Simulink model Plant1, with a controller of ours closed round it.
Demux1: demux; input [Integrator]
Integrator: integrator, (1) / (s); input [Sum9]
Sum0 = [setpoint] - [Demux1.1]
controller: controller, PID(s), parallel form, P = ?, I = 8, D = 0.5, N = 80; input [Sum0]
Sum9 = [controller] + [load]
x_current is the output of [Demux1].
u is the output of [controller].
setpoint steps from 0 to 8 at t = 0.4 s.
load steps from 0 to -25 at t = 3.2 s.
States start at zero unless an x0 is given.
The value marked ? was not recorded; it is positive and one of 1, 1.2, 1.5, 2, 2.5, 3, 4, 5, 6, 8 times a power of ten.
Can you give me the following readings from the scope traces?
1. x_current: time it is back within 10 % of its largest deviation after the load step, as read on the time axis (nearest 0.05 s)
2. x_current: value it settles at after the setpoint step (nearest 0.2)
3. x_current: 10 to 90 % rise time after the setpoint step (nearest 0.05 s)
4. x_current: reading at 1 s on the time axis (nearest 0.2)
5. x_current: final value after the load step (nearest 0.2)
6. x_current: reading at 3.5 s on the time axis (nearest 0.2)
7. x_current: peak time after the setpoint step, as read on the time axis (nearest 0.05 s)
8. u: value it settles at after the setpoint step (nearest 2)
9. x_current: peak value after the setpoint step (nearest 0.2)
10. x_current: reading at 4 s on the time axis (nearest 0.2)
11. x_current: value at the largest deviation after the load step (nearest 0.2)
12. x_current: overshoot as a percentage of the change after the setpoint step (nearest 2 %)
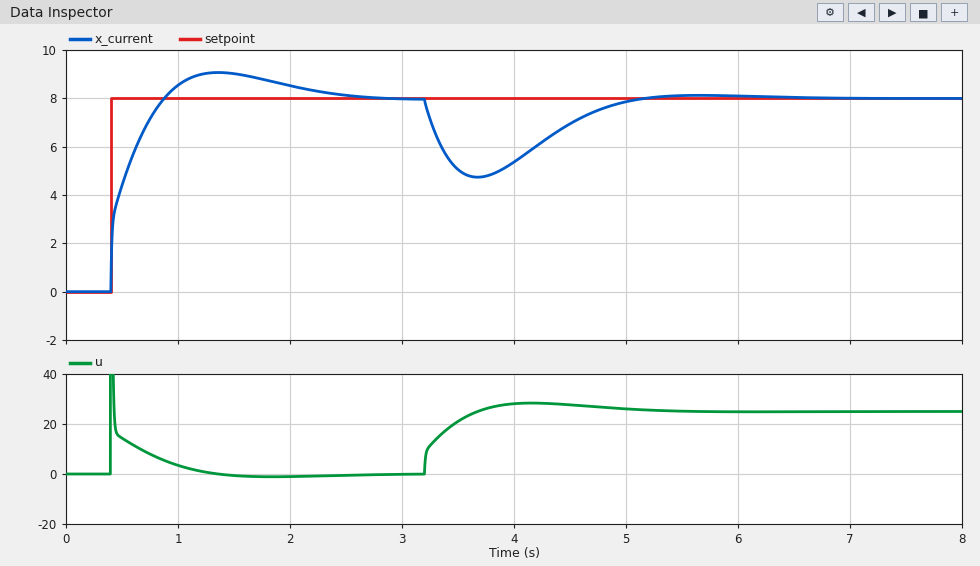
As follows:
4.85 s
8.0
0.35 s
8.6
8.0
5.0
1.35 s
0
9.0
5.4
4.8
14 %
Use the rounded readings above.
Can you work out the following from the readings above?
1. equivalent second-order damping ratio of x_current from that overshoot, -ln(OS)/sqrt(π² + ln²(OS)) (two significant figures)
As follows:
0.53
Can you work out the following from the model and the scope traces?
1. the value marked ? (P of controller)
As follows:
5
